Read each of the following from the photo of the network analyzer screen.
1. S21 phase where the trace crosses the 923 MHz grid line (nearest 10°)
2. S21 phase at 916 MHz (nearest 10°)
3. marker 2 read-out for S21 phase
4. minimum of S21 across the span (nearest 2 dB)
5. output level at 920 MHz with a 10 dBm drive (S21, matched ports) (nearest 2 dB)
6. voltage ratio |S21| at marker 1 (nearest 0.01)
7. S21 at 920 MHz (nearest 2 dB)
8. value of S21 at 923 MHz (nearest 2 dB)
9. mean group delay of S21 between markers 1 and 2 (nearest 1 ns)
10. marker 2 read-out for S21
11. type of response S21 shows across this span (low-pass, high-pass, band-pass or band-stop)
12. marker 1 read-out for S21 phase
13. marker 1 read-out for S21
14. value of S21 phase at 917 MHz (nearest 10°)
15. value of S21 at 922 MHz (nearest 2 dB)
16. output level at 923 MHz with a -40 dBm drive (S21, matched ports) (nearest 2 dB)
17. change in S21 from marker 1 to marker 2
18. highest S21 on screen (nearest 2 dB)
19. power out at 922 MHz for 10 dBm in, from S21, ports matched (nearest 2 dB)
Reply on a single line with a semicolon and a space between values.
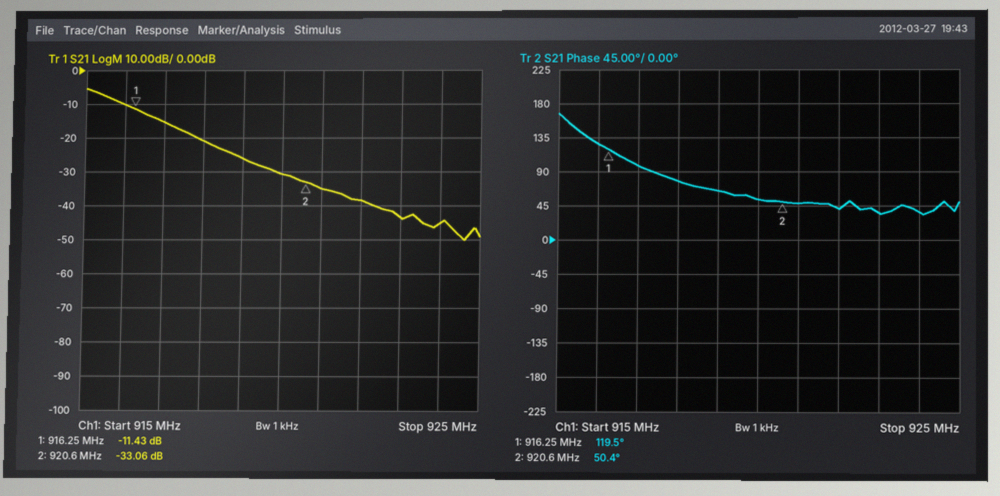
40°; 130°; 50.4°; -50 dB; -20 dBm; 0.27; -30 dB; -44 dB; 44 ns; -33.06 dB; low-pass; 119.5°; -11.43 dB; 100°; -38 dB; -84 dBm; -21.63 dB; -6 dB; -28 dBm
